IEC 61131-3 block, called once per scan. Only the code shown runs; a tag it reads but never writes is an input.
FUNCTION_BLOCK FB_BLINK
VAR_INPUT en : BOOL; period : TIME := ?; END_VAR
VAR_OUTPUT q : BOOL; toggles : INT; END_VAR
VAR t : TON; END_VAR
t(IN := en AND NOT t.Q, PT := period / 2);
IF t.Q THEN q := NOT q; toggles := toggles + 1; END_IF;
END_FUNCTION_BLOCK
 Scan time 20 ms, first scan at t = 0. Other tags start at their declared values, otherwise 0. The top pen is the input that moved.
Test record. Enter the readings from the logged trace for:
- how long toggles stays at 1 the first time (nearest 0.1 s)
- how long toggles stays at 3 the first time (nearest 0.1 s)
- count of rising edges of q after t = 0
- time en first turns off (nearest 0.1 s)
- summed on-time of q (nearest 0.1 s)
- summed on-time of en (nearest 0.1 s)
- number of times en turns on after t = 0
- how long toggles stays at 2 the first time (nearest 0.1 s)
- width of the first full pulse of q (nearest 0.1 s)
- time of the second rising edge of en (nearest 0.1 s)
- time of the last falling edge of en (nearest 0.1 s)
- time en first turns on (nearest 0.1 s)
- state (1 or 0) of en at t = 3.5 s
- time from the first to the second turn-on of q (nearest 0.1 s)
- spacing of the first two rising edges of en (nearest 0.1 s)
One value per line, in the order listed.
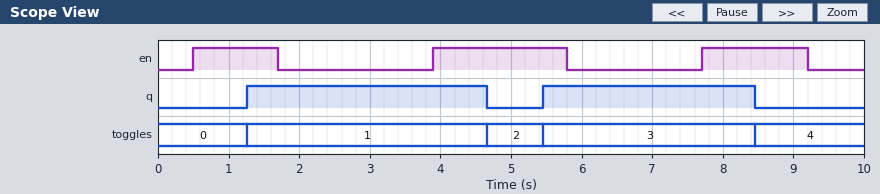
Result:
3.4 s
3.0 s
2
1.7 s
6.4 s
4.6 s
3
0.8 s
3.4 s
3.9 s
9.2 s
0.5 s
0
4.2 s
3.4 s
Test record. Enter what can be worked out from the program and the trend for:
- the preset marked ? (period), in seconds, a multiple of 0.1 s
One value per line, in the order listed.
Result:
1.5 s
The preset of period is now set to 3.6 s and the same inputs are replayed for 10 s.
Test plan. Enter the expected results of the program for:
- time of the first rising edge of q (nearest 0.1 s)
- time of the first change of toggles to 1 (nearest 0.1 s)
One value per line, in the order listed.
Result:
5.7 s
5.7 s
